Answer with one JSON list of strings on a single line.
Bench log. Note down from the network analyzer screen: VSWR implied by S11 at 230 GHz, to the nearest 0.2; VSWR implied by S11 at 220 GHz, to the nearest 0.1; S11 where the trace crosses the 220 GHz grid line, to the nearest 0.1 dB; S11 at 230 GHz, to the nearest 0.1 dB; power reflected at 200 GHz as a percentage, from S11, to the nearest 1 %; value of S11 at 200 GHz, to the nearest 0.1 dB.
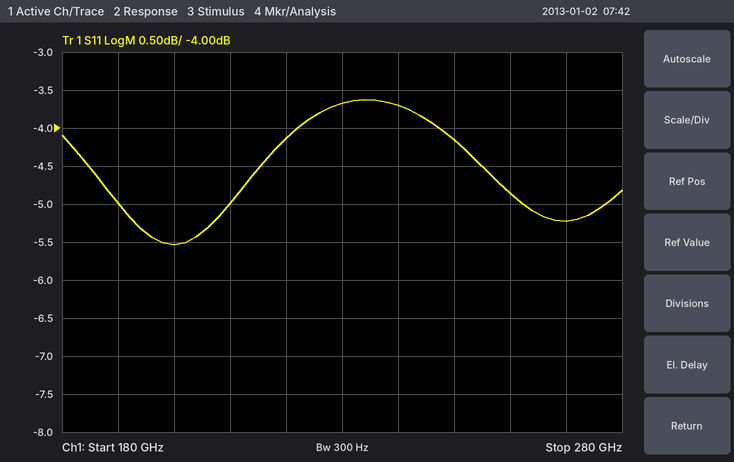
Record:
["4.8", "4.3", "-4.1 dB", "-3.7 dB", "28 %", "-5.5 dB"]
